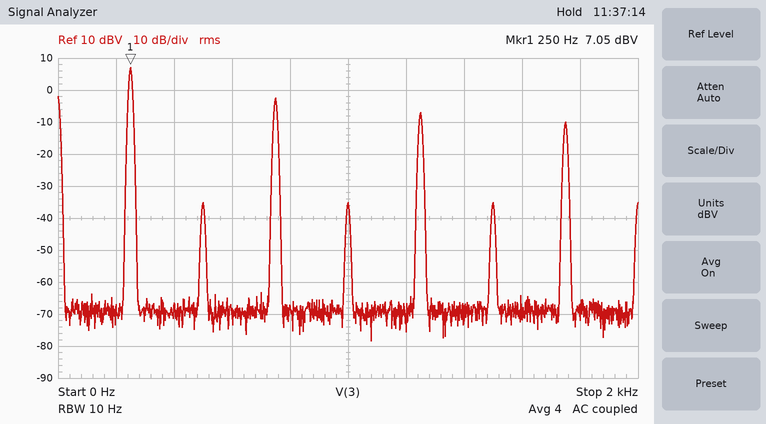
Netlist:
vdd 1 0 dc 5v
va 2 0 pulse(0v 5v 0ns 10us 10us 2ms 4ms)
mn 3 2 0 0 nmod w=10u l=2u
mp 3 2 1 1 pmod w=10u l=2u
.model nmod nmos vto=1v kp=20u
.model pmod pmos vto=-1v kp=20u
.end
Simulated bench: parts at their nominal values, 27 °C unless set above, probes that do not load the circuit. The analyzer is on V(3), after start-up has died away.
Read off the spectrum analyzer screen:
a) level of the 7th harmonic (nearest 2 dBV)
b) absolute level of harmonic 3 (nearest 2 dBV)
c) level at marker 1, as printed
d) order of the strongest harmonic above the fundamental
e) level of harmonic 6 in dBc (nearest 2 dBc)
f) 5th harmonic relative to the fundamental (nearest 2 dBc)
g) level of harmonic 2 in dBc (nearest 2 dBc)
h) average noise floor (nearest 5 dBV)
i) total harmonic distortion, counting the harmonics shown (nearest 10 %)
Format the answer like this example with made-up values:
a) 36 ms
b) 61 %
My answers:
a) -10 dBV
b) -2 dBV
c) 7.05 dBV
d) 3
e) -42 dBc
f) -14 dBc
g) -42 dBc
h) -70 dBV
i) 40 %
